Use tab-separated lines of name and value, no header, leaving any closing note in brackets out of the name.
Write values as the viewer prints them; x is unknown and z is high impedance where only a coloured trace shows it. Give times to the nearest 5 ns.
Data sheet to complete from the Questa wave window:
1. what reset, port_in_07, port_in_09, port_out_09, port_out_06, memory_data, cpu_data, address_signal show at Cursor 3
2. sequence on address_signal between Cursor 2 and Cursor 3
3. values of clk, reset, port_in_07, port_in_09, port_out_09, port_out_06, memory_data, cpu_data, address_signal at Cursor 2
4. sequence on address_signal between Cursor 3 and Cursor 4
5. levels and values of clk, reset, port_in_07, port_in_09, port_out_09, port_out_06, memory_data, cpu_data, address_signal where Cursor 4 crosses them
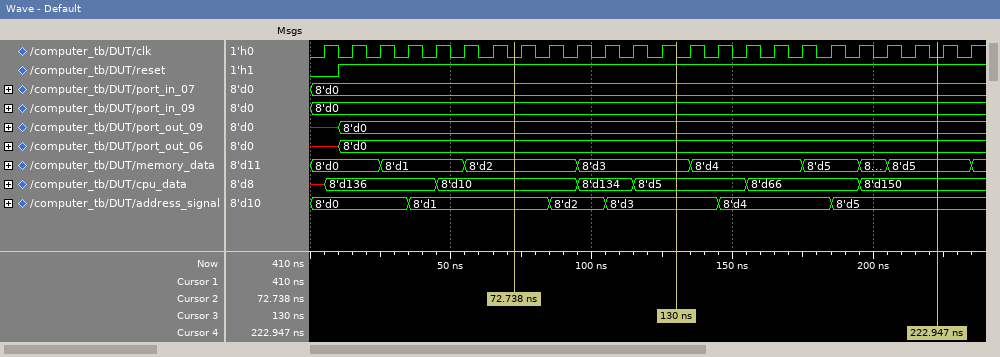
what reset, port_in_07, port_in_09, port_out_09, port_out_06, memory_data, cpu_data, address_signal show at Cursor 3	reset=1, port_in_07=8'd0, port_in_09=8'd0, port_out_09=8'd0, port_out_06=8'd0, memory_data=8'd3, cpu_data=8'd5, address_signal=8'd3
sequence on address_signal between Cursor 2 and Cursor 3	8'd1, 8'd2, 8'd3
values of clk, reset, port_in_07, port_in_09, port_out_09, port_out_06, memory_data, cpu_data, address_signal at Cursor 2	clk=0, reset=1, port_in_07=8'd0, port_in_09=8'd0, port_out_09=8'd0, port_out_06=8'd0, memory_data=8'd2, cpu_data=8'd10, address_signal=8'd1
sequence on address_signal between Cursor 3 and Cursor 4	8'd3, 8'd4, 8'd5
levels and values of clk, reset, port_in_07, port_in_09, port_out_09, port_out_06, memory_data, cpu_data, address_signal where Cursor 4 crosses them	clk=0, reset=1, port_in_07=8'd0, port_in_09=8'd0, port_out_09=8'd0, port_out_06=8'd0, memory_data=8'd5, cpu_data=8'd150, address_signal=8'd5
